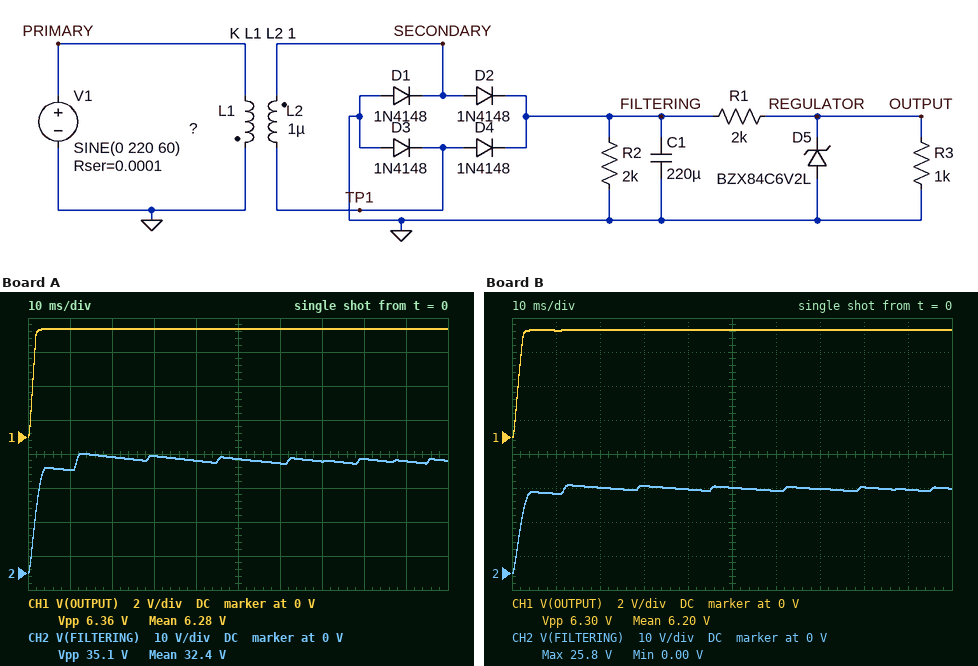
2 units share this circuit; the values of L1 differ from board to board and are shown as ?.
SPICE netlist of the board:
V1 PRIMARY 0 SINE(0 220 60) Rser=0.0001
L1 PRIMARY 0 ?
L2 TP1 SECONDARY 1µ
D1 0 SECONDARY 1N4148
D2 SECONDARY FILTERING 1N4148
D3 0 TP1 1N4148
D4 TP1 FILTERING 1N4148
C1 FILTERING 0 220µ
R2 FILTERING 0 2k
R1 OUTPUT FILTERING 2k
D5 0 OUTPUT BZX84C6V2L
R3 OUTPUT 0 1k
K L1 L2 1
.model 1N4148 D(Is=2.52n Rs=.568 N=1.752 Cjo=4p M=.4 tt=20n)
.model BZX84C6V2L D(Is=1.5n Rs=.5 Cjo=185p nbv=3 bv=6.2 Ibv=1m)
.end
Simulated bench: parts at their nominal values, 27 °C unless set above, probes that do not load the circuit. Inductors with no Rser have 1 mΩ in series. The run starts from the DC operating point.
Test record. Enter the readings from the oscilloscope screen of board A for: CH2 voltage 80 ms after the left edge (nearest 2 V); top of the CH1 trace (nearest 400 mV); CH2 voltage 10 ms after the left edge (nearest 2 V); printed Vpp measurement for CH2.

34 V
6.4 V
30 V
35.1 V
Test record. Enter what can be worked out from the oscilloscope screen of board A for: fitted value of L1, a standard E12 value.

39 µH
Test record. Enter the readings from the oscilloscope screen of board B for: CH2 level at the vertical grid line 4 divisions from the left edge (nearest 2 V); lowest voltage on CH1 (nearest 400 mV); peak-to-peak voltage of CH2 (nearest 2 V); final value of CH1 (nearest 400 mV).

24 V
0 V
26 V
6.4 V
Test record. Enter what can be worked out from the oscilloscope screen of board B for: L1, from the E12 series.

68 µH
